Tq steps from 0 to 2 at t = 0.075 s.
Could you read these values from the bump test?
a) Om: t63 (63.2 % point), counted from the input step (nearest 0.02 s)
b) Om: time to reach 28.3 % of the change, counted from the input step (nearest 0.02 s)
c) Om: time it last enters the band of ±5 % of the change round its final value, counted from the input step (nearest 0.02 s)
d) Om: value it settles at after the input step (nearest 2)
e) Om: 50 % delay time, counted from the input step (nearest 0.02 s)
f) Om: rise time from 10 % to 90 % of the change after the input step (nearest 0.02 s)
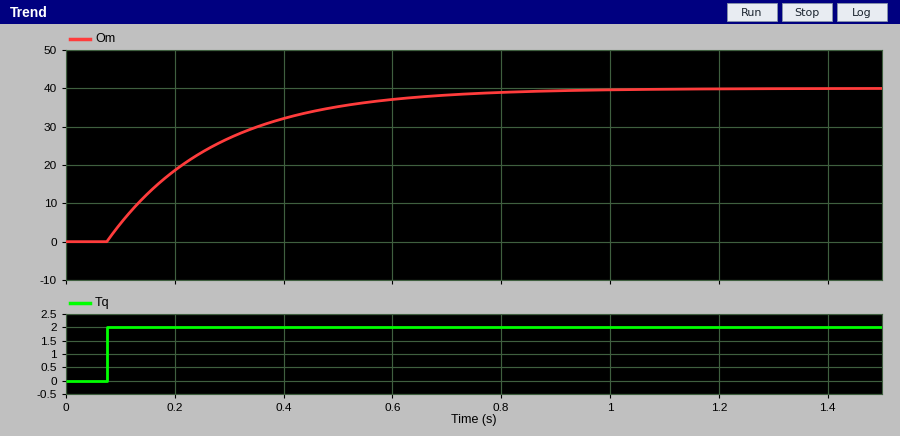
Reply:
0.20 s
0.06 s
0.60 s
40
0.14 s
0.44 s
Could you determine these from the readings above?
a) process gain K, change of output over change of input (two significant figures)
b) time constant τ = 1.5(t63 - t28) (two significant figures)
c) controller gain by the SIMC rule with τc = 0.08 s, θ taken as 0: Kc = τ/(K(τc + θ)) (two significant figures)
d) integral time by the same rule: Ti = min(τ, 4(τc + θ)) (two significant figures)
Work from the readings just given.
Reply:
20
0.21 s
0.13
0.21 s
